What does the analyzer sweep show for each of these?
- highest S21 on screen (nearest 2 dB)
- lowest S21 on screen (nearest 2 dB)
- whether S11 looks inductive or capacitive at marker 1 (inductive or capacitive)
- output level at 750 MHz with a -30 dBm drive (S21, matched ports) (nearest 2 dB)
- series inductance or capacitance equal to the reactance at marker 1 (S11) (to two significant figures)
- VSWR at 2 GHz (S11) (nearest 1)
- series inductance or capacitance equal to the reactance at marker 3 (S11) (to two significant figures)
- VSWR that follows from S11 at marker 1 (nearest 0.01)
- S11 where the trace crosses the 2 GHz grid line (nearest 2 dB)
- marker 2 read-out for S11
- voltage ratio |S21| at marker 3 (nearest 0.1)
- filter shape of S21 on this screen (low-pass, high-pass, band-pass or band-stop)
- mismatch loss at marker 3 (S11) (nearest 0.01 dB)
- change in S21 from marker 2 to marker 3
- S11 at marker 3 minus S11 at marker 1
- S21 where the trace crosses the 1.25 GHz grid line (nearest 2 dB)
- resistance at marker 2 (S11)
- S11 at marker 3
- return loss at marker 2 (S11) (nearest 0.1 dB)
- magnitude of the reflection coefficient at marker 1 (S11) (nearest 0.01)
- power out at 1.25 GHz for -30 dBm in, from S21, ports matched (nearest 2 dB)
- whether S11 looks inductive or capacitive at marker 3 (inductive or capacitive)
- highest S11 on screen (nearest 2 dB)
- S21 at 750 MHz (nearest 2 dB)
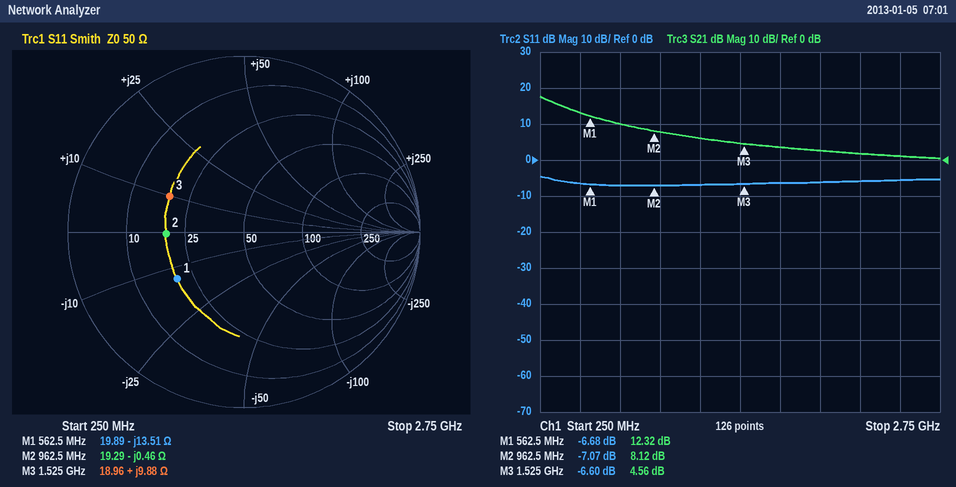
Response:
18 dB
0 dB
capacitive
-20 dBm
21 pF
3
1.0 nH
2.73
-6 dB
-7.07 dB
1.7
low-pass
1.07 dB
-3.56 dB
0.08 dB
6 dB
19.29 Ω
-6.60 dB
7.1 dB
0.46
-24 dBm
inductive
-4 dB
10 dB
